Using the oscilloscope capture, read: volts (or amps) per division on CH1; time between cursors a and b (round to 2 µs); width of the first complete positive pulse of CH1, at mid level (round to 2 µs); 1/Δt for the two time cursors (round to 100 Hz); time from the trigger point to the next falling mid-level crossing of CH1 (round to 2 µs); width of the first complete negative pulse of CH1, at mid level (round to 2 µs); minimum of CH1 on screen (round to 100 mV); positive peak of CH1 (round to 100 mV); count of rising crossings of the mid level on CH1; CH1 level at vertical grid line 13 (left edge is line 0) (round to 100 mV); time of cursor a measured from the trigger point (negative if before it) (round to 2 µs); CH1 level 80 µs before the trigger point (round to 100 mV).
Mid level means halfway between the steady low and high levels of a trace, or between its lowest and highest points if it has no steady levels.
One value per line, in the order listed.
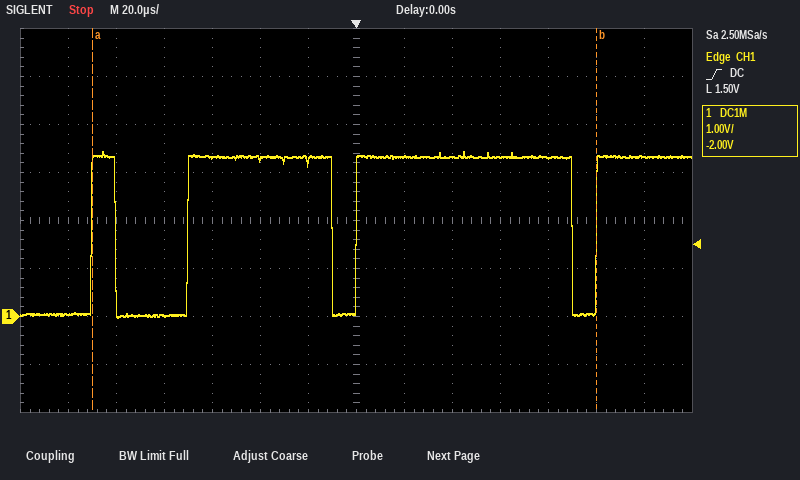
1 V
210 µs
10 µs
4.8 kHz
90 µs
30 µs
0.0 V
3.4 V
4
3.3 V
-110 µs
0.0 V
